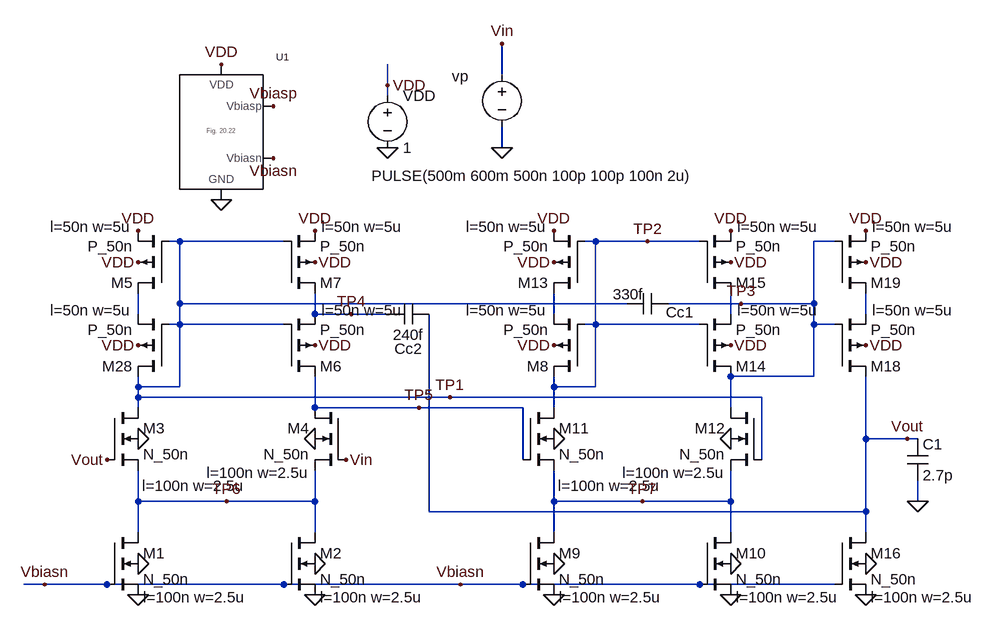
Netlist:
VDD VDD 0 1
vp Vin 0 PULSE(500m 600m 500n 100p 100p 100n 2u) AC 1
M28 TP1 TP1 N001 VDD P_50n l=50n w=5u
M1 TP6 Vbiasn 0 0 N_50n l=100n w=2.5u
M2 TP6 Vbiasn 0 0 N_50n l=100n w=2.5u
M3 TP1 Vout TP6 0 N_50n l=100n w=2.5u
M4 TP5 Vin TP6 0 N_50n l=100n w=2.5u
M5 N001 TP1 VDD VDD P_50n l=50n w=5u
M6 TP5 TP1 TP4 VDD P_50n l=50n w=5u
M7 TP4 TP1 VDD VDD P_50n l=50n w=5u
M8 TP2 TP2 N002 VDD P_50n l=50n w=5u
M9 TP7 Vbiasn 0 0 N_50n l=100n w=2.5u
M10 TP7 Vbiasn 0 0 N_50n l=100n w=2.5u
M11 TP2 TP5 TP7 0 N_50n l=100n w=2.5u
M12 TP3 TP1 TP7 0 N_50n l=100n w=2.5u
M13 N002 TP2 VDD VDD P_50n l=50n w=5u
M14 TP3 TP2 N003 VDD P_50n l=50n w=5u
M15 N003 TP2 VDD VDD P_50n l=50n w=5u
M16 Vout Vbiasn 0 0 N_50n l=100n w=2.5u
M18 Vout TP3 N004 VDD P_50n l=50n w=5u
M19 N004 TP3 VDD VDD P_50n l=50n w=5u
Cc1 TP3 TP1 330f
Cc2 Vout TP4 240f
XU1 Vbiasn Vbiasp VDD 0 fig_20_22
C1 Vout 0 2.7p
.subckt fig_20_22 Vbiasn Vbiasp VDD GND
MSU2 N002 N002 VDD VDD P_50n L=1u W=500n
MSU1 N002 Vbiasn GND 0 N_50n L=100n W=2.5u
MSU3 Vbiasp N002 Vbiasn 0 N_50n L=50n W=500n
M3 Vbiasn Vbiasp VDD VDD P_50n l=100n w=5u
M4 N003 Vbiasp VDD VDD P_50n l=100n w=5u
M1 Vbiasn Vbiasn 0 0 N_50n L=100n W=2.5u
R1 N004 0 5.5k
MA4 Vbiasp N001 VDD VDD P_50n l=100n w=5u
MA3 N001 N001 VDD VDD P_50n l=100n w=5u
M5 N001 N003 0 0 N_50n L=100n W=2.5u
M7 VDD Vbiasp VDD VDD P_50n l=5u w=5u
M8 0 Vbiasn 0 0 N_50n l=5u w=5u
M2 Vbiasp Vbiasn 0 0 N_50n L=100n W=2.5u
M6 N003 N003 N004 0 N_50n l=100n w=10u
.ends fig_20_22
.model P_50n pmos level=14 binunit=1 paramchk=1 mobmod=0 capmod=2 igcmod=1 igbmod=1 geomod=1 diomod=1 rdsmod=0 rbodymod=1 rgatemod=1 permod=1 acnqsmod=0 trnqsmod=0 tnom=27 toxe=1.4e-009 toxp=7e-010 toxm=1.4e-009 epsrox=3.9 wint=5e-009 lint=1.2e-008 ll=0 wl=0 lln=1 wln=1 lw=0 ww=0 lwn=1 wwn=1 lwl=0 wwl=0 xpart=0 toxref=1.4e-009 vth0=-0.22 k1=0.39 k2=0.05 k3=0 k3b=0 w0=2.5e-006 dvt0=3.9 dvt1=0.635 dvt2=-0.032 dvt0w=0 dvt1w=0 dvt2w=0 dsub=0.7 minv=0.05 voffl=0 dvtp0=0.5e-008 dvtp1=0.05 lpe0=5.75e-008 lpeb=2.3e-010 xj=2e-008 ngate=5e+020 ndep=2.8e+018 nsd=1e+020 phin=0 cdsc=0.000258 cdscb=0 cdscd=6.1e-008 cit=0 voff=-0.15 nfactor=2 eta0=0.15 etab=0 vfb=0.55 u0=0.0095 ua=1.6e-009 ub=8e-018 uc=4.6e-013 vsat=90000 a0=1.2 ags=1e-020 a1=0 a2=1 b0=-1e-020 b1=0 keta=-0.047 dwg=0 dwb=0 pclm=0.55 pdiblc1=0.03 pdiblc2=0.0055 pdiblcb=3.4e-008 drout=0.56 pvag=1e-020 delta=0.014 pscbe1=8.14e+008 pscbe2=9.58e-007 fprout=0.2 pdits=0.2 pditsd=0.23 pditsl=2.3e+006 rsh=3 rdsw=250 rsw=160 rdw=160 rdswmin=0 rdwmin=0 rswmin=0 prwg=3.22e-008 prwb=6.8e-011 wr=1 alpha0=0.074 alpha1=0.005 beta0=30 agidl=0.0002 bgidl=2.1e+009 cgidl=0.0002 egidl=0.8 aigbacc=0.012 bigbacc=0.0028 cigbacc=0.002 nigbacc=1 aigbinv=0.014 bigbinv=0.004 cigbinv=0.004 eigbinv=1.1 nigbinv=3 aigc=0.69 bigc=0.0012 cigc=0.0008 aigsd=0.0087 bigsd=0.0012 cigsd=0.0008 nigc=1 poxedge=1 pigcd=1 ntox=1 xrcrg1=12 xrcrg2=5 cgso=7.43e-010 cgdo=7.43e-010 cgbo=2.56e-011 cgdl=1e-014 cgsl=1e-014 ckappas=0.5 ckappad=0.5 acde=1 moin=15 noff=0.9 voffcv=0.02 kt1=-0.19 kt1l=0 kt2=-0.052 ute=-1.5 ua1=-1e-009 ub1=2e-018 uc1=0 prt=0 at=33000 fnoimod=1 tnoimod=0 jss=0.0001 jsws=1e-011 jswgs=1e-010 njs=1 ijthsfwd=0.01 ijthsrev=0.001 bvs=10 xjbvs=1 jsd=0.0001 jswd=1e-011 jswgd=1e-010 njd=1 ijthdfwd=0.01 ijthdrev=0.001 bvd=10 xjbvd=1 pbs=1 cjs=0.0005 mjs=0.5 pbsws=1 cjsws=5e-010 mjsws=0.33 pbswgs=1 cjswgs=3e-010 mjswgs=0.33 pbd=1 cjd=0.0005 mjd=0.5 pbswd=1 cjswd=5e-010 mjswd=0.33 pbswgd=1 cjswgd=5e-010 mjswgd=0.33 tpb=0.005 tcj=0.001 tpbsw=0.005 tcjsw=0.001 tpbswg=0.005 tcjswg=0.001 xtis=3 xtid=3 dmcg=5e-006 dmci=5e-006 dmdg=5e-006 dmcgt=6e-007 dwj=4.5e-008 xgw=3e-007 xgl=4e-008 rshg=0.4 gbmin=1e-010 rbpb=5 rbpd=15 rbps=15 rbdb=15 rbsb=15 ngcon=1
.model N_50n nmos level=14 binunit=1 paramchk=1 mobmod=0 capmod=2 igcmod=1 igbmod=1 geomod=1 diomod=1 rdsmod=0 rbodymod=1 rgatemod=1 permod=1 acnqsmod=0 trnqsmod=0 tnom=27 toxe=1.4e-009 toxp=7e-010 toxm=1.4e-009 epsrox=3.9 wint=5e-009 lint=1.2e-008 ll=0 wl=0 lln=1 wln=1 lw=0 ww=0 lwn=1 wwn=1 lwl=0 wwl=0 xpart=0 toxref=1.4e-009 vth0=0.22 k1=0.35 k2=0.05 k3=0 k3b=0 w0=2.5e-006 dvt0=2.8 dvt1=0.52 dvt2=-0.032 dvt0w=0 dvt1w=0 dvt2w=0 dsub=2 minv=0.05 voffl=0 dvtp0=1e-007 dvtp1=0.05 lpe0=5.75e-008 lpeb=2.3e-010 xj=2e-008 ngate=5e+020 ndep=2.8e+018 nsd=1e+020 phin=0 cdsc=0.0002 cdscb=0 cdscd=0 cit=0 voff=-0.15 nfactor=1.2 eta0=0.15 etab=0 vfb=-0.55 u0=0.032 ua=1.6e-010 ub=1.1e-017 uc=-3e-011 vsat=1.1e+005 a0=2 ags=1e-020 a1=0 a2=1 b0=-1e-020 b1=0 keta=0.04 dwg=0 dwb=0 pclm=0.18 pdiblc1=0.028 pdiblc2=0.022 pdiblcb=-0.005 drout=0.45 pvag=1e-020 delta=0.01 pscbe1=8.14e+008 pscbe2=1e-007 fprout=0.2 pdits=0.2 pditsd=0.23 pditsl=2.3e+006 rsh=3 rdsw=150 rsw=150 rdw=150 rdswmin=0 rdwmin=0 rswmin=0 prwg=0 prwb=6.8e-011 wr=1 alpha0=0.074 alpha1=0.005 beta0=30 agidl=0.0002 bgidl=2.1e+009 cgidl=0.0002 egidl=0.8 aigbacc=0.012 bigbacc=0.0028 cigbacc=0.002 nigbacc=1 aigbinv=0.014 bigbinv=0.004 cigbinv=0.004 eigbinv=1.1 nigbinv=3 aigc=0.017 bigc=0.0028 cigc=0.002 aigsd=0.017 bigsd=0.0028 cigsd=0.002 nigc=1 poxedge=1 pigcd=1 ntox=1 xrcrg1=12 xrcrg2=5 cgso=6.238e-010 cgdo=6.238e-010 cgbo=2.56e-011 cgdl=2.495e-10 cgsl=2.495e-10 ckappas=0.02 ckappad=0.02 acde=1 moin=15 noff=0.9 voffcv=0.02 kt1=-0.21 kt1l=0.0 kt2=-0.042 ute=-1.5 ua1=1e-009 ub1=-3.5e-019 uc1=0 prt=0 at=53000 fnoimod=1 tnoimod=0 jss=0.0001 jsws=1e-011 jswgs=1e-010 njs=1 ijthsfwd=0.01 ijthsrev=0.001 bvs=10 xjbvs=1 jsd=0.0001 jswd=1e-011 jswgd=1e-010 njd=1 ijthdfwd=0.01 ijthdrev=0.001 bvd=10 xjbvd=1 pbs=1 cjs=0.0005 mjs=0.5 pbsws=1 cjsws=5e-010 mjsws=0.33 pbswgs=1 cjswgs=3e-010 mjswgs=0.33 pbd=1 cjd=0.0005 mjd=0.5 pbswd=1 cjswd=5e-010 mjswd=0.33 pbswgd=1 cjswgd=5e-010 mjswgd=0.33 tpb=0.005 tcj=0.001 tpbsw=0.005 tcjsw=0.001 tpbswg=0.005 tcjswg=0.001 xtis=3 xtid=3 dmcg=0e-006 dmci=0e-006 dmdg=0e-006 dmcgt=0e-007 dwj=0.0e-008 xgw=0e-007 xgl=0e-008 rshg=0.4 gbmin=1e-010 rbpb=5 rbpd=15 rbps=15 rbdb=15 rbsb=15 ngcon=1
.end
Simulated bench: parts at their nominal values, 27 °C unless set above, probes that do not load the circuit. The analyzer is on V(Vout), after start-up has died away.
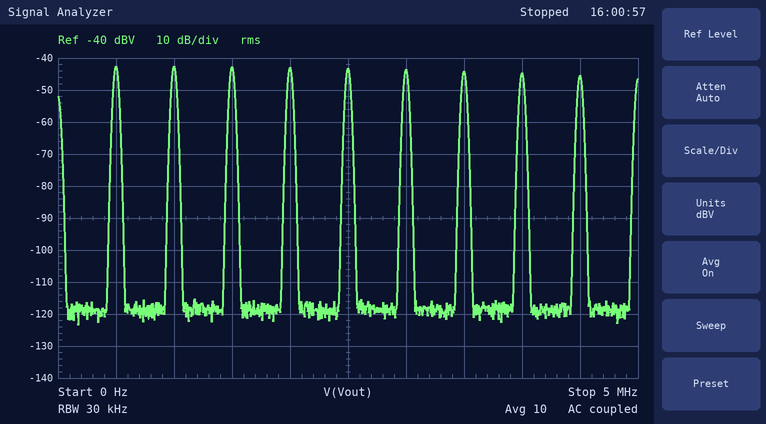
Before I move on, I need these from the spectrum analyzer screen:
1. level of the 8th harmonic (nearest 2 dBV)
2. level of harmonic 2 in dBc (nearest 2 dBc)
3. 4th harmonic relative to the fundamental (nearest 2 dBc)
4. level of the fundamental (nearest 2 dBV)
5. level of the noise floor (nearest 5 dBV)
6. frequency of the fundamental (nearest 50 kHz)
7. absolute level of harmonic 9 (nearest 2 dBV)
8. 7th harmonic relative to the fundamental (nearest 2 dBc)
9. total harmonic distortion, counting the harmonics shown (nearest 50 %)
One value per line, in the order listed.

-44 dBV
0 dBc
0 dBc
-42 dBV
-120 dBV
500 kHz
-46 dBV
-2 dBc
250 %
